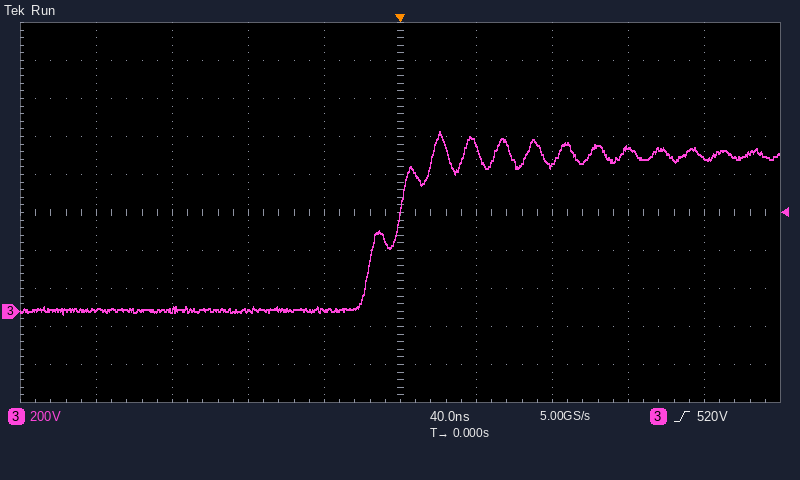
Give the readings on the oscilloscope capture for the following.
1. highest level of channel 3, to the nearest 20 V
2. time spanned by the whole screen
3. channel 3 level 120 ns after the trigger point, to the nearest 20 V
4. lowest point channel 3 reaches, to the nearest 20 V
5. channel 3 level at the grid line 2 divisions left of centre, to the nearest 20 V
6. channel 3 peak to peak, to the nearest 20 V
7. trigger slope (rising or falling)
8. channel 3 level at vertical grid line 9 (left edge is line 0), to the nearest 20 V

940 V
400 ns
860 V
-20 V
0 V
960 V
rising
800 V
